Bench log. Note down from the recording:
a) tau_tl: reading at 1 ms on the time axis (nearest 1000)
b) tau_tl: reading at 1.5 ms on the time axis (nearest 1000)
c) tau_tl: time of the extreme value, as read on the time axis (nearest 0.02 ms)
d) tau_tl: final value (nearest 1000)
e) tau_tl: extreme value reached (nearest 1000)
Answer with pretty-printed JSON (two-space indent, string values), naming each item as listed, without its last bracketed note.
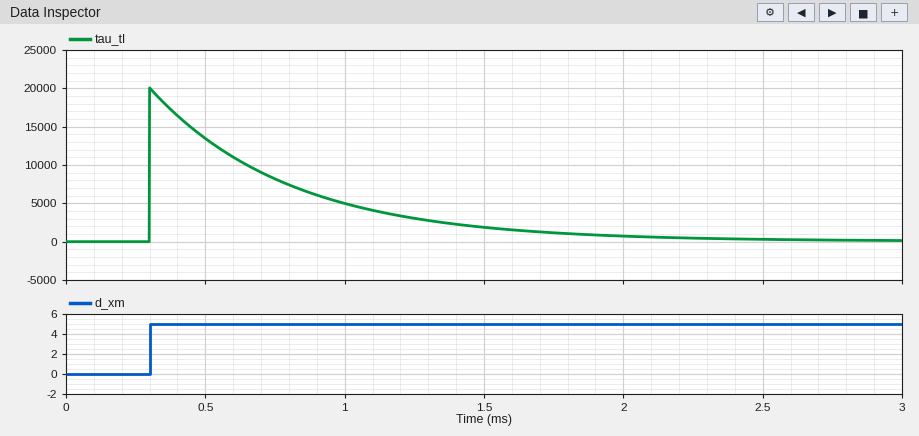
{
  "tau_tl: reading at 1 ms on the time axis": "5000",
  "tau_tl: reading at 1.5 ms on the time axis": "2000",
  "tau_tl: time of the extreme value, as read on the time axis": "0.30 ms",
  "tau_tl: final value": "0",
  "tau_tl: extreme value reached": "20000"
}
